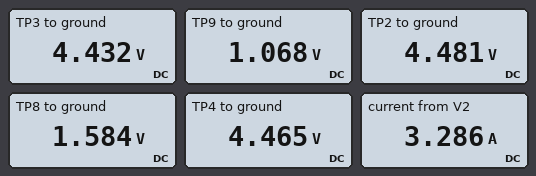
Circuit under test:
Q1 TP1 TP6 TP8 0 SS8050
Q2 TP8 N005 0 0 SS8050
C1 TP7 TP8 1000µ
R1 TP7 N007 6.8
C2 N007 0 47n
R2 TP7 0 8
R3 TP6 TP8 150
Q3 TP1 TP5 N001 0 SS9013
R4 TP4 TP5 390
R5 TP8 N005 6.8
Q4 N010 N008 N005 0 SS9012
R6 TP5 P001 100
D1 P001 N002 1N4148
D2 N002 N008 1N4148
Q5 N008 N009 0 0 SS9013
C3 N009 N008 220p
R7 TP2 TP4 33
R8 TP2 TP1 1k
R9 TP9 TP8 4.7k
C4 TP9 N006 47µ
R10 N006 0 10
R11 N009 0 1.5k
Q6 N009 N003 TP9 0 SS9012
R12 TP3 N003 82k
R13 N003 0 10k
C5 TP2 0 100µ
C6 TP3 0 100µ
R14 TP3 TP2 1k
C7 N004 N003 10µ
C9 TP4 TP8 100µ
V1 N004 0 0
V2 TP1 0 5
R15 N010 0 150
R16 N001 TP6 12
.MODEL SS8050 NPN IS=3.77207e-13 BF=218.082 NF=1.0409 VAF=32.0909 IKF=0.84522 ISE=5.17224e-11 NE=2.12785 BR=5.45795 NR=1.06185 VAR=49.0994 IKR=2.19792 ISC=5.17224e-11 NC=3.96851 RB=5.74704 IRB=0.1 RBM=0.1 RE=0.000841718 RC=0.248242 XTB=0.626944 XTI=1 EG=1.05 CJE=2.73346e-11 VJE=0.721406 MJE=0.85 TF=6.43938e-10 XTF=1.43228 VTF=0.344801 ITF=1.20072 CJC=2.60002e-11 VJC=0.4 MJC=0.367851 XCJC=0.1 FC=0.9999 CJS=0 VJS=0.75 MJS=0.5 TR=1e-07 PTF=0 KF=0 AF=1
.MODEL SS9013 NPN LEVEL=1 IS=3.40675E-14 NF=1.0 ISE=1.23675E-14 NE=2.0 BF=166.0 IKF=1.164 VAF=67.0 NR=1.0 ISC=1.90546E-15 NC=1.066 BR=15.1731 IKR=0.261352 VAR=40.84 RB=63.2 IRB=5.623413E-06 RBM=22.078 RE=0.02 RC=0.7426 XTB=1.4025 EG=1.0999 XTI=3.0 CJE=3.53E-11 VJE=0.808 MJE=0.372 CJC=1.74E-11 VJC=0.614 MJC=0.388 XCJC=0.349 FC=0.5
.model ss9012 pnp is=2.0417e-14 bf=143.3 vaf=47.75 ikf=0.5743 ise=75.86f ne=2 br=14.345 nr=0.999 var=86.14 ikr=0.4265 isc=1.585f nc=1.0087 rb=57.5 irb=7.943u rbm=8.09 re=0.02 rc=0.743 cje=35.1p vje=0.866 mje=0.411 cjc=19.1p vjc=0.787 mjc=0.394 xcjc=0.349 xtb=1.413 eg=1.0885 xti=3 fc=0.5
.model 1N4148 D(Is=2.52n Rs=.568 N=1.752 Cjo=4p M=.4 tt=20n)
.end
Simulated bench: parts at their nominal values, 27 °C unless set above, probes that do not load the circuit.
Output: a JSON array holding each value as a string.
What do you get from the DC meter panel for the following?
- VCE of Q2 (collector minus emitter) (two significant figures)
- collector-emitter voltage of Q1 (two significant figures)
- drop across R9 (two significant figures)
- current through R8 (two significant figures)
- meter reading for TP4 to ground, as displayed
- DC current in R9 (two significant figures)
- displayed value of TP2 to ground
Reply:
["1.6 V", "3.4 V", "520 mV", "520 µA", "4.465 V", "110 µA", "4.481 V"]
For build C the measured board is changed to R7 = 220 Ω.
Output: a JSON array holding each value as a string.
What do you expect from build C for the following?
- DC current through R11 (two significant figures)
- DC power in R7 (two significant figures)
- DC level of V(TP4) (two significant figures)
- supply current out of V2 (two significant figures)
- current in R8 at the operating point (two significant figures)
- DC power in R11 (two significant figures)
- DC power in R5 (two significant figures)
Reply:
["100 µA", "45 µW", "4.4 V", "3.2 A", "500 µA", "16 µW", "34 mW"]
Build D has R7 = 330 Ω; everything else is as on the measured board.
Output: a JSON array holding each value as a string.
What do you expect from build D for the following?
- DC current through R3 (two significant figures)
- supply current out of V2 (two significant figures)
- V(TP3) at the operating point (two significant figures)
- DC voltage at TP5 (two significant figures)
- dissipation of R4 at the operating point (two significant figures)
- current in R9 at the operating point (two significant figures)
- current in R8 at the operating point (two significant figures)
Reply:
["7.0 mA", "3.2 A", "4.5 V", "4.2 V", "77 µW", "100 µA", "490 µA"]
